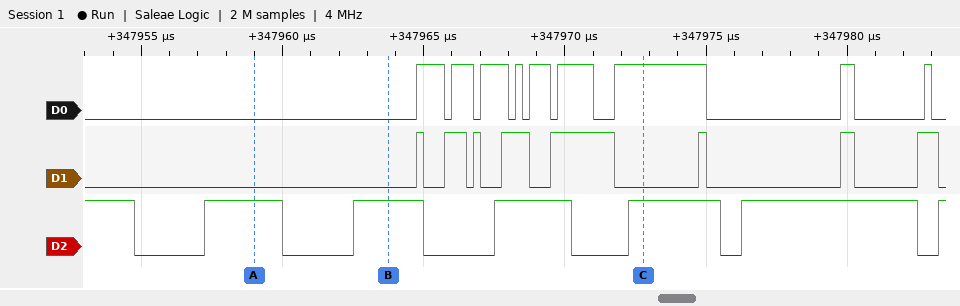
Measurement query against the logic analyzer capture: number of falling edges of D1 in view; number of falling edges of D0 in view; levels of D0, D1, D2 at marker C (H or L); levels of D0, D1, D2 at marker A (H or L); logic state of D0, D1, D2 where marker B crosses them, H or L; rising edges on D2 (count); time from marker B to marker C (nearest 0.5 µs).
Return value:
8
9
D0=H, D1=L, D2=H
D0=L, D1=L, D2=H
D0=L, D1=L, D2=H
6
9 µs
